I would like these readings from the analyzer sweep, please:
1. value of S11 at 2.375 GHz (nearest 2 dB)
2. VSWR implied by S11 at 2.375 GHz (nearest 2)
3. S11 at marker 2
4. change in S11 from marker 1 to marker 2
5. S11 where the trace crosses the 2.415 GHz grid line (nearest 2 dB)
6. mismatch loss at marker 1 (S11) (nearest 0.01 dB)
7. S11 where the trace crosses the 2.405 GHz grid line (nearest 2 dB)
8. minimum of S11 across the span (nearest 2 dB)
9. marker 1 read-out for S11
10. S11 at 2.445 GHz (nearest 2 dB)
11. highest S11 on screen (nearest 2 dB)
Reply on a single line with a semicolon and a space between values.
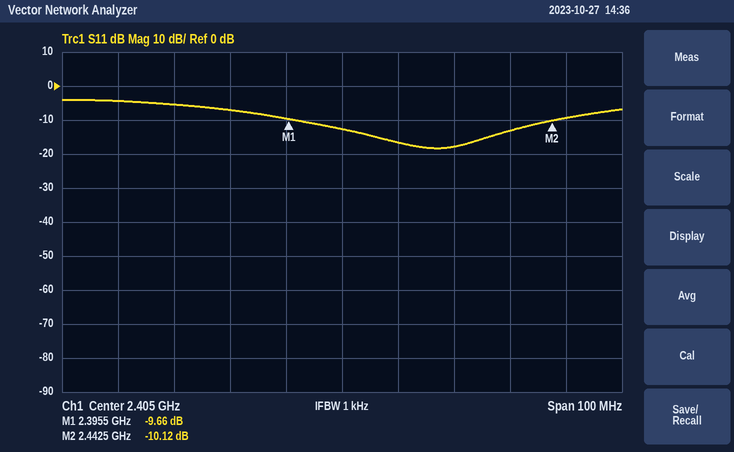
-6 dB; 4; -10.12 dB; -0.46 dB; -16 dB; 0.50 dB; -12 dB; -18 dB; -9.66 dB; -10 dB; -4 dB
